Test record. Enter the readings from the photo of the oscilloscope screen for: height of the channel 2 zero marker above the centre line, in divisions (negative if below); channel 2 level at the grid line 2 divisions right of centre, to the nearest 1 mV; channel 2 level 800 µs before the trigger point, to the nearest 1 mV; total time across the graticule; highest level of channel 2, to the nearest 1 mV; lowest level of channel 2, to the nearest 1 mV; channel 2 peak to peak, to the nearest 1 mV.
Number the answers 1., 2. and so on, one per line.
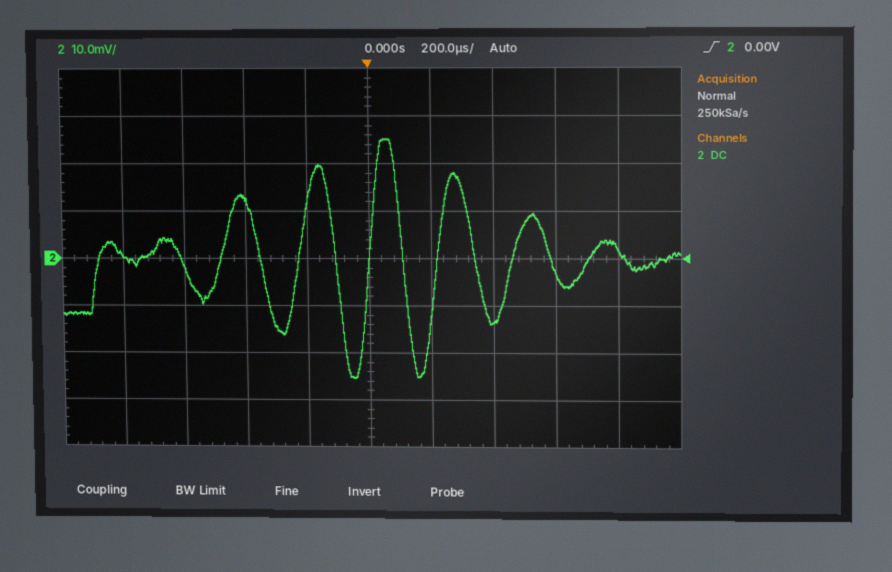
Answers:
1. 0.0 div
2. -13 mV
3. 1 mV
4. 2 ms
5. 25 mV
6. -25 mV
7. 50 mV
